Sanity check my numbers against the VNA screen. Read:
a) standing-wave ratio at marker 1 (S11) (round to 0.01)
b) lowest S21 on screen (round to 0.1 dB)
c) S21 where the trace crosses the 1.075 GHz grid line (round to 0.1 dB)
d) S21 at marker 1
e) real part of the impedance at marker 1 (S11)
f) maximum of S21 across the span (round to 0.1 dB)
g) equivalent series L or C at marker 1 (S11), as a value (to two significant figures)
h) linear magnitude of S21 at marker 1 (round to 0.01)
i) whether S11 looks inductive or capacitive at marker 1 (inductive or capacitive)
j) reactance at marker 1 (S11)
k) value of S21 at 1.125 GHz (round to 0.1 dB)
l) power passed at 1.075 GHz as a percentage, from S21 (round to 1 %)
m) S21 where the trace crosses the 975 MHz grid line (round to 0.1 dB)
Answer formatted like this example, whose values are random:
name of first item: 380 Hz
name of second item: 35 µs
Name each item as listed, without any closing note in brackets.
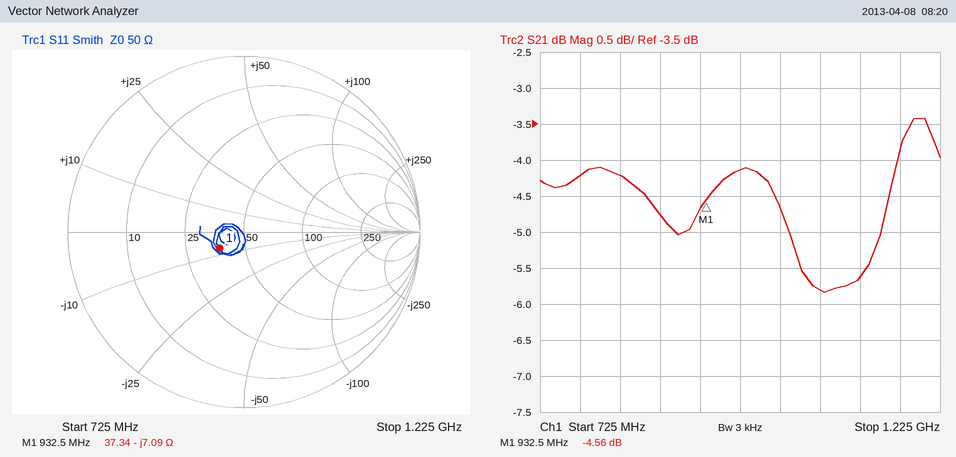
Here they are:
standing-wave ratio at marker 1 (S11): 1.40
lowest S21 on screen: -5.8 dB
S21 where the trace crosses the 1.075 GHz grid line: -5.8 dB
S21 at marker 1: -4.56 dB
real part of the impedance at marker 1: 37.34 Ω
maximum of S21 across the span: -3.4 dB
equivalent series L or C at marker 1 (S11), as a value: 24 pF
linear magnitude of S21 at marker 1: 0.59
whether S11 looks inductive or capacitive at marker 1: capacitive
reactance at marker 1: -7.09 Ω
value of S21 at 1.125 GHz: -5.6 dB
power passed at 1.075 GHz as a percentage, from S21: 26 %
S21 where the trace crosses the 975 MHz grid line: -4.1 dB
